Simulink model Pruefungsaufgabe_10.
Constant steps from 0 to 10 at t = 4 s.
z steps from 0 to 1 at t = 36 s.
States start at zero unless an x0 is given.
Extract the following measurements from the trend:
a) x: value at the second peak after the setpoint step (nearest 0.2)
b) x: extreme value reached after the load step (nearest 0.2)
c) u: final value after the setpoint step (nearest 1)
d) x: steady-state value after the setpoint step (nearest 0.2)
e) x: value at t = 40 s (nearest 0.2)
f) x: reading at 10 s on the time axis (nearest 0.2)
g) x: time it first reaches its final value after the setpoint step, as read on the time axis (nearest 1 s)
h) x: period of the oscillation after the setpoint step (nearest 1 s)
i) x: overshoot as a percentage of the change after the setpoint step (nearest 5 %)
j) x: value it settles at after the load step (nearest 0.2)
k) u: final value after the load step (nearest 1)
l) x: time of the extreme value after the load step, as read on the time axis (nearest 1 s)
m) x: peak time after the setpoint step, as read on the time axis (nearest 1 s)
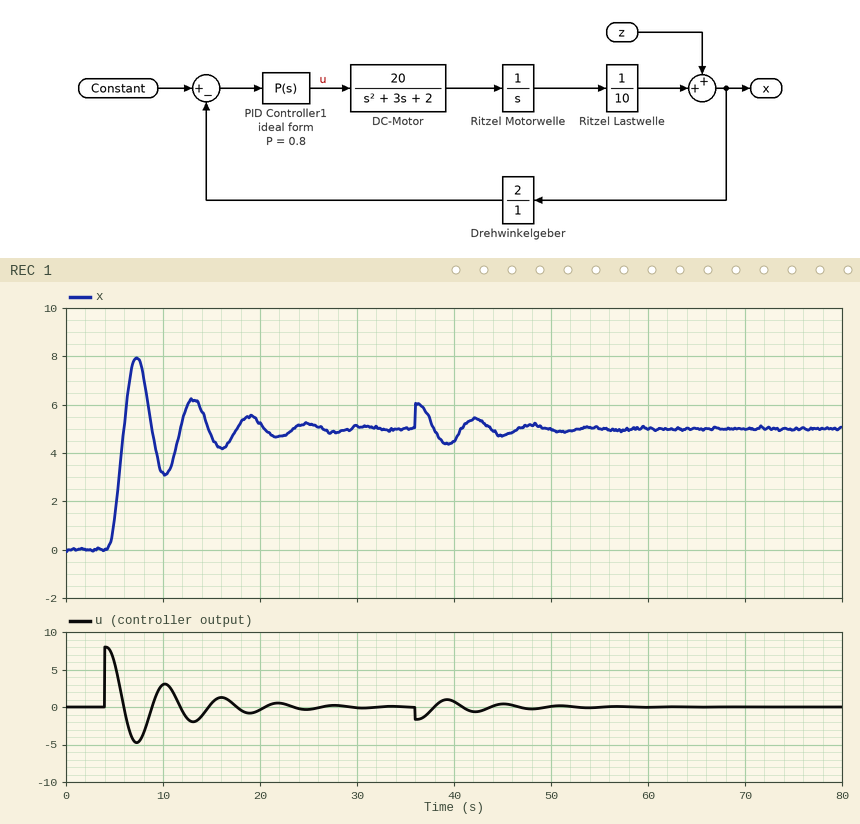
6.2
6.0
0
5.0
4.6
3.2
6 s
6 s
60 %
5.0
0
36 s
7 s
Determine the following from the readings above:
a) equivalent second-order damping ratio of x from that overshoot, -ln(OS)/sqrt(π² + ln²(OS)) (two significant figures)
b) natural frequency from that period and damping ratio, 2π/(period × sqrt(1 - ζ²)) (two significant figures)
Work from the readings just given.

0.16
1.1 rad/s
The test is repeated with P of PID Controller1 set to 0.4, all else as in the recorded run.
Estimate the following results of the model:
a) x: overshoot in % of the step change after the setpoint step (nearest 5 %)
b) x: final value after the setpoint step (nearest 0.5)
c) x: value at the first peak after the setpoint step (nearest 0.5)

30 %
5.0
6.5
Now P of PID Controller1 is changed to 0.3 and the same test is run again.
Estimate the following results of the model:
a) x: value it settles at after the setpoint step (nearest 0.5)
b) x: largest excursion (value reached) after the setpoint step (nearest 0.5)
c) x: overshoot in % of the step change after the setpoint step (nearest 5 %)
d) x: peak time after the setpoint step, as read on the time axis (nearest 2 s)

5.0
6.0
20 %
10 s
